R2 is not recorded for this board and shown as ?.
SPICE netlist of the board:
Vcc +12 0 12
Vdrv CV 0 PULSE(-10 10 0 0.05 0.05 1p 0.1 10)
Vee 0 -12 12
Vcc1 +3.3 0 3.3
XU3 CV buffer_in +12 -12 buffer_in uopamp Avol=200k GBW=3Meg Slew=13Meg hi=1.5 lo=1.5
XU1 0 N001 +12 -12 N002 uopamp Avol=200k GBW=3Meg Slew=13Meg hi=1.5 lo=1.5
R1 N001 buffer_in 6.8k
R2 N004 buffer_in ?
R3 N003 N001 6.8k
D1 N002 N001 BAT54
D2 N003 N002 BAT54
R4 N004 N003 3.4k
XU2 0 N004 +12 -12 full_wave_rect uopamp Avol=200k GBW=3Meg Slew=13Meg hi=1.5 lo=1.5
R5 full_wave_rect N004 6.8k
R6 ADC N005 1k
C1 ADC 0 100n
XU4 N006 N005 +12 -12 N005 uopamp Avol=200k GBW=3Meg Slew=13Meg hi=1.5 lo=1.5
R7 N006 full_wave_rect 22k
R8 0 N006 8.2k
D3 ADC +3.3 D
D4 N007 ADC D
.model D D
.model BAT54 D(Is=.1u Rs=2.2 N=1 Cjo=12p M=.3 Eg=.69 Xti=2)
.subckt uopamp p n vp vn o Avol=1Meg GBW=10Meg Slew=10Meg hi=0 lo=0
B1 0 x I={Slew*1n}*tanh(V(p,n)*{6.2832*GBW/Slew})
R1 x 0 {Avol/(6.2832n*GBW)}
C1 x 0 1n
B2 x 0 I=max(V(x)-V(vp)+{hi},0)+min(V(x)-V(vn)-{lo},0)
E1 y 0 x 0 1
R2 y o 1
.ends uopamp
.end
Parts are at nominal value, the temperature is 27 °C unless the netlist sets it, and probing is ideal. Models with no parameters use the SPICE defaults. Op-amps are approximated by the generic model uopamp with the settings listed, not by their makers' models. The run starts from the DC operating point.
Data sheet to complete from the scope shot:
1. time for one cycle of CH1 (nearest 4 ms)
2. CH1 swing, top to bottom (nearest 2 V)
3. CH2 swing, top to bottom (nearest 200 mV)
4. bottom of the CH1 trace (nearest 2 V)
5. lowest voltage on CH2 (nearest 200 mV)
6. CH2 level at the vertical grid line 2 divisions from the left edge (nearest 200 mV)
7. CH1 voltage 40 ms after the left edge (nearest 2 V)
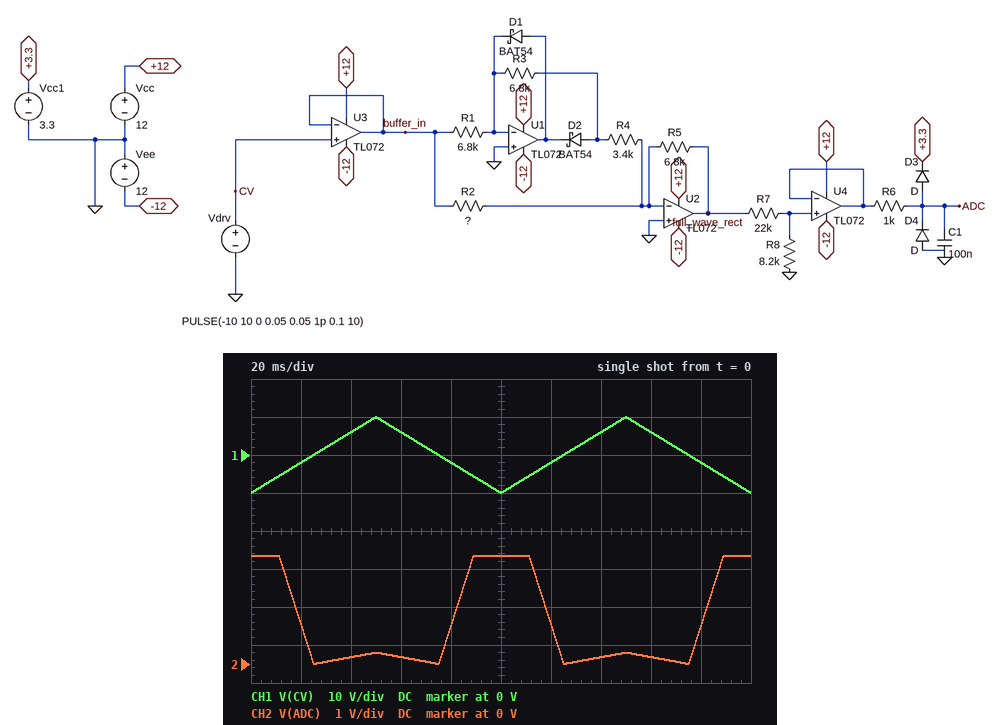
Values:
100 ms
20 V
2.8 V
-10 V
0 V
200 mV
6 V
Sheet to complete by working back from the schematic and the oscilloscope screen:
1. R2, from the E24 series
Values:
3.6 kΩ
